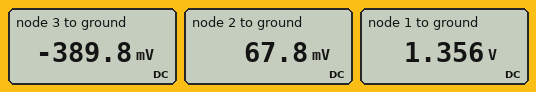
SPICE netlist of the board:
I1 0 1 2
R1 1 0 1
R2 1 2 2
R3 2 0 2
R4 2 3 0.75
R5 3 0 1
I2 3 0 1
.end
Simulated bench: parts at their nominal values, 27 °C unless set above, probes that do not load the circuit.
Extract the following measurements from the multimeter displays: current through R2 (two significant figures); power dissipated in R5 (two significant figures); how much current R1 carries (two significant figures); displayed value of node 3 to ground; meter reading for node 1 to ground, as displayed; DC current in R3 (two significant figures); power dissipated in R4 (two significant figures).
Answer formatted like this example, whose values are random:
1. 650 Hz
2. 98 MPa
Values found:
1. 640 mA
2. 150 mW
3. 1.4 A
4. -389.8 mV
5. 1.356 V
6. 34 mA
7. 280 mW
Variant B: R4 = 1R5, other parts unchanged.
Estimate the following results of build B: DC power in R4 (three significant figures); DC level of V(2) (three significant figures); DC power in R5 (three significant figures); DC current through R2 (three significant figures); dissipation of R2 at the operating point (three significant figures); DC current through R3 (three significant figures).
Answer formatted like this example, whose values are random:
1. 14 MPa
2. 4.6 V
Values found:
1. 355 mW
2. 216 mV
3. 264 mW
4. 595 mA
5. 707 mW
6. 108 mA
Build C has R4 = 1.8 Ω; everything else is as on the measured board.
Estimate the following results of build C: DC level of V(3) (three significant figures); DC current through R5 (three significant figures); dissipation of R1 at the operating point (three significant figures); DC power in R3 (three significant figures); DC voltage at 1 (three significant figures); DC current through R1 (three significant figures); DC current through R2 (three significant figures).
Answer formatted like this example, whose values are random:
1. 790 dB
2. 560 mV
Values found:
1. -550 mV
2. 550 mA
3. 2.02 W
4. 33.8 mW
5. 1.42 V
6. 1.42 A
7. 580 mA
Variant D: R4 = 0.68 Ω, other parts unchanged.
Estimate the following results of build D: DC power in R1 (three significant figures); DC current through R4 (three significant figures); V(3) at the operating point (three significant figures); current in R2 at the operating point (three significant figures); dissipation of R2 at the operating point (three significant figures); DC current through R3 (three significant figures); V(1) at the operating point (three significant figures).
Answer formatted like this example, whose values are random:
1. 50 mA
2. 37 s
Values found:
1. 1.82 W
2. 625 mA
3. -375 mV
4. 650 mA
5. 845 mW
6. 25.0 mA
7. 1.35 V
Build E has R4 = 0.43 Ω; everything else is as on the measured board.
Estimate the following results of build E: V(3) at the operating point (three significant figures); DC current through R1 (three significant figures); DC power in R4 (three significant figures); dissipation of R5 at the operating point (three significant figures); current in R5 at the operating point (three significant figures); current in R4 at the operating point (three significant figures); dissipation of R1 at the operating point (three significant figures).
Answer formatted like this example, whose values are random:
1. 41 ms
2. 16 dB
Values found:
1. -316 mV
2. 1.33 A
3. 201 mW
4. 99.6 mW
5. 316 mA
6. 684 mA
7. 1.76 W
